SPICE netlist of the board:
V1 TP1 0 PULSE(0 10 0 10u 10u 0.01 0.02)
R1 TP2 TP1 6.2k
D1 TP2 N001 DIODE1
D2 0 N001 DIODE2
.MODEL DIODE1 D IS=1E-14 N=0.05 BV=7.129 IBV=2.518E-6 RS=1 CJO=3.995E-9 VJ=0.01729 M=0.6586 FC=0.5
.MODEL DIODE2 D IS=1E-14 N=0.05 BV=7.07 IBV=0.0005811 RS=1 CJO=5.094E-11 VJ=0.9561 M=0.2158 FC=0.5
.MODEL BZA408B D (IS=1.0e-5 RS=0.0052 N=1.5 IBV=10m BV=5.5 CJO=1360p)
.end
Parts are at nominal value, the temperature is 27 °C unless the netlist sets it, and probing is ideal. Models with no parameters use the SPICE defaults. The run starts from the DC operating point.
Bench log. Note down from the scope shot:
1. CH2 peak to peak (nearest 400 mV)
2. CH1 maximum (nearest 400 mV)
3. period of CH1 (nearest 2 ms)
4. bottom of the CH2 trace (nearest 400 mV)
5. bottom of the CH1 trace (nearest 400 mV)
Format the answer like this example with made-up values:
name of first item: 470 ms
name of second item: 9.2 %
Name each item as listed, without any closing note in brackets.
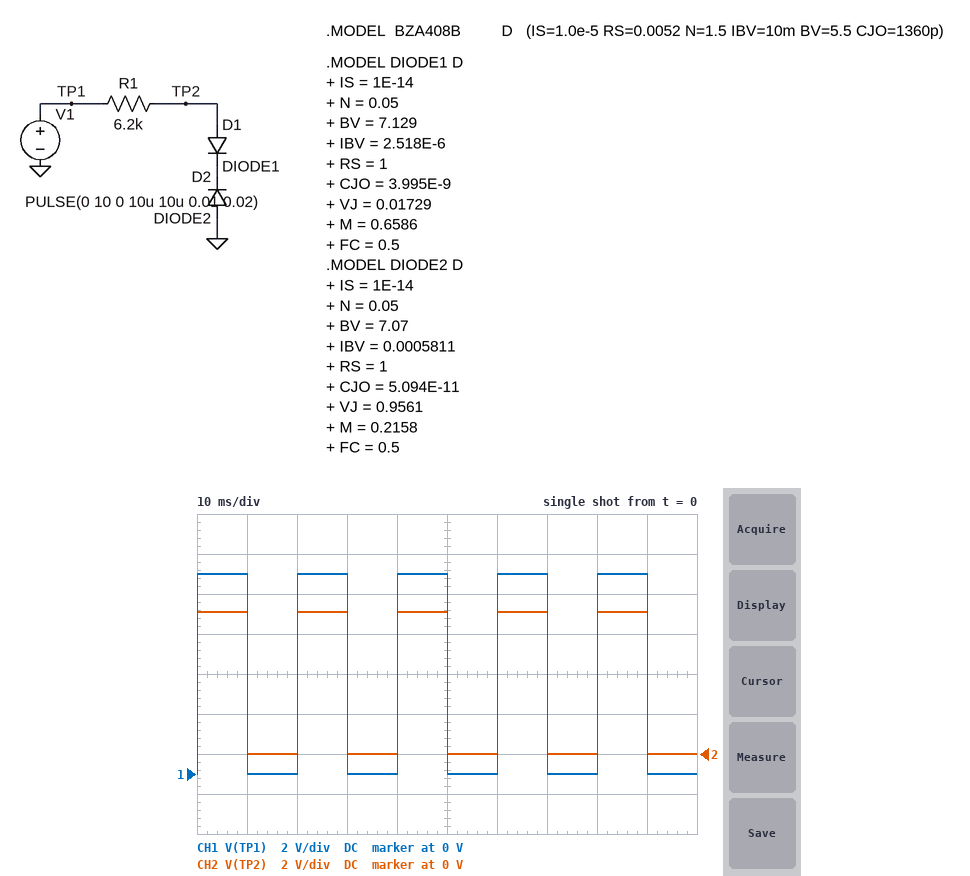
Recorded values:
CH2 peak to peak: 7.2 V
CH1 maximum: 10.0 V
period of CH1: 20 ms
bottom of the CH2 trace: 0 V
bottom of the CH1 trace: 0 V
